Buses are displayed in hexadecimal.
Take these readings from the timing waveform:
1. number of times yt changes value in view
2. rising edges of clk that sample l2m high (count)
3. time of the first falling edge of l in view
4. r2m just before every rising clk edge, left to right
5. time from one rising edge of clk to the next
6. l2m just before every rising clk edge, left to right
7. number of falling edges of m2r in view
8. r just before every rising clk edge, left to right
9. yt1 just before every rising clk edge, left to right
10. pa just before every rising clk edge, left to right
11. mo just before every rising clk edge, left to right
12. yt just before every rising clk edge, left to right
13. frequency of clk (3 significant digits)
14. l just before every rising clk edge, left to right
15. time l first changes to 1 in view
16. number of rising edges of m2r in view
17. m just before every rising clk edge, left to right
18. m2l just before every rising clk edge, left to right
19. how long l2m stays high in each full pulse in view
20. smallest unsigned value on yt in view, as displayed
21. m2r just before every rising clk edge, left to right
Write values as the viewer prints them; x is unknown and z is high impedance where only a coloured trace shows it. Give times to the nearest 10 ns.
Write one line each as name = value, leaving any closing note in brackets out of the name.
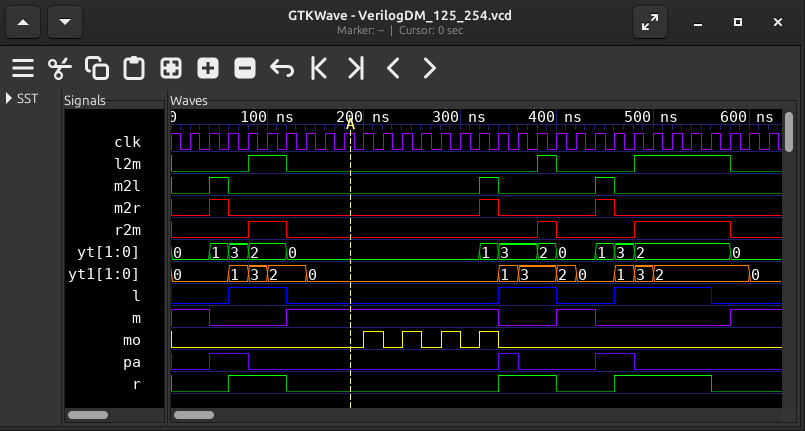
number of times yt changes value in view = 12
rising edges of clk that sample l2m high = 8
time of the first falling edge of l in view = 120 ns
r2m just before every rising clk edge, left to right = 0 0 0 0 1 1 0 0 0 0 0 0 0 0 0 0 0 0 0 1 0 0 0 0 1 1 1 1 1 0 0
time from one rising edge of clk to the next = 20 ns
l2m just before every rising clk edge, left to right = 0 0 0 0 1 1 0 0 0 0 0 0 0 0 0 0 0 0 0 1 0 0 0 0 1 1 1 1 1 0 0
number of falling edges of m2r in view = 3
r just before every rising clk edge, left to right = 0 0 0 1 1 1 0 0 0 0 0 0 0 0 0 0 0 1 1 1 0 0 0 1 1 1 1 1 0 0 0
yt1 just before every rising clk edge, left to right = 0, 0, 0, 1, 3, 2, 2, 0, 0, 0, 0, 0, 0, 0, 0, 0, 0, 1, 3, 3, 2, 0, 0, 1, 3, 2, 2, 2, 2, 2, 0
pa just before every rising clk edge, left to right = 0 0 1 1 0 0 0 0 0 0 0 0 0 0 0 0 0 1 0 0 0 0 1 1 0 0 0 0 0 0 0
mo just before every rising clk edge, left to right = 0 0 0 0 0 0 0 0 0 0 1 0 1 0 1 0 1 0 0 0 0 0 0 0 0 0 0 0 0 0 0
yt just before every rising clk edge, left to right = 0, 0, 1, 3, 2, 2, 0, 0, 0, 0, 0, 0, 0, 0, 0, 0, 1, 3, 3, 2, 0, 0, 1, 3, 2, 2, 2, 2, 2, 0, 0
frequency of clk = 50.0 MHz
l just before every rising clk edge, left to right = 0 0 0 1 1 1 0 0 0 0 0 0 0 0 0 0 0 1 1 1 0 0 0 1 1 1 1 1 0 0 0
time l first changes to 1 in view = 60 ns
number of rising edges of m2r in view = 3
m just before every rising clk edge, left to right = 1 1 0 0 0 0 1 1 1 1 1 1 1 1 1 1 1 0 0 0 1 1 0 0 0 0 0 0 0 1 1
m2l just before every rising clk edge, left to right = 0 0 1 0 0 0 0 0 0 0 0 0 0 0 0 0 1 0 0 0 0 0 1 0 0 0 0 0 0 0 0
how long l2m stays high in each full pulse in view = 40 ns, 20 ns, 100 ns
smallest unsigned value on yt in view, as displayed = 0
m2r just before every rising clk edge, left to right = 0 0 1 0 0 0 0 0 0 0 0 0 0 0 0 0 1 0 0 0 0 0 1 0 0 0 0 0 0 0 0
